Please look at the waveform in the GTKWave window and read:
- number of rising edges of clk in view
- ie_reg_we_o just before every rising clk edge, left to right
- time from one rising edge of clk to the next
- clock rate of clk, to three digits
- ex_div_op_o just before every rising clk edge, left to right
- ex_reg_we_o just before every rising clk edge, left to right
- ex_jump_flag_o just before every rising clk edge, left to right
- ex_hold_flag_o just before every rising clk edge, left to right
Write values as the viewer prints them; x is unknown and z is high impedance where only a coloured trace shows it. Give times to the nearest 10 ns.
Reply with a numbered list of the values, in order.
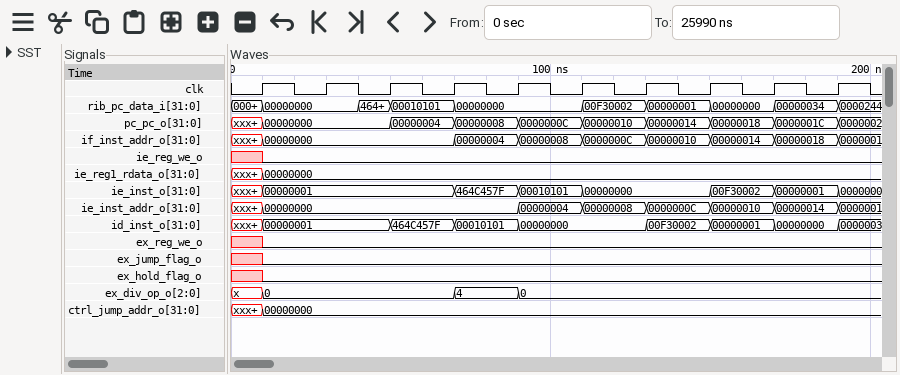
1. 10
2. x 0 0 0 0 0 0 0 0 0
3. 20 ns
4. 50.0 MHz
5. x, 0, 0, 0, 4, 0, 0, 0, 0, 0
6. x 0 0 0 0 0 0 0 0 0
7. x 0 0 0 0 0 0 0 0 0
8. x 0 0 0 0 0 0 0 0 0
